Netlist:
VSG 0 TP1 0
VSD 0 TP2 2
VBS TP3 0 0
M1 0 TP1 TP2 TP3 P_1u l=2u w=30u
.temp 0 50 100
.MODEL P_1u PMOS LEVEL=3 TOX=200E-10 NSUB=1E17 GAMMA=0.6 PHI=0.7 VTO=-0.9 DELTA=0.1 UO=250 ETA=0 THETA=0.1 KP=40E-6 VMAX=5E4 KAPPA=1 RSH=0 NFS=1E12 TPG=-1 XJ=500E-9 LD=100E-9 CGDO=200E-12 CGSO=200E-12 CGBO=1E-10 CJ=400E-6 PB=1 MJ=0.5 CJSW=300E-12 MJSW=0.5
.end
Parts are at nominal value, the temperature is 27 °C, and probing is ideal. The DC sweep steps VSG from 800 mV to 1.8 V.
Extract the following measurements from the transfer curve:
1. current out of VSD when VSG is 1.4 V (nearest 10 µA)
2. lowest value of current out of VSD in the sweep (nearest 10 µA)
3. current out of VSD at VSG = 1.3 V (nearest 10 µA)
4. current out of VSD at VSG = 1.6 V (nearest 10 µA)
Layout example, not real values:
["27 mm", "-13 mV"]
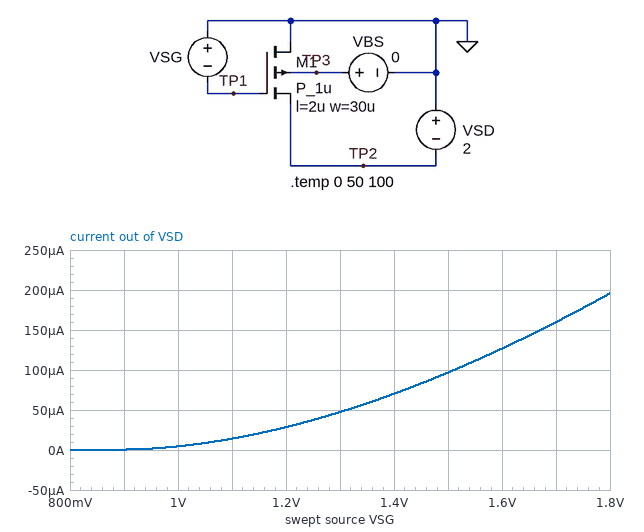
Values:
["70 µA", "0 A", "50 µA", "130 µA"]
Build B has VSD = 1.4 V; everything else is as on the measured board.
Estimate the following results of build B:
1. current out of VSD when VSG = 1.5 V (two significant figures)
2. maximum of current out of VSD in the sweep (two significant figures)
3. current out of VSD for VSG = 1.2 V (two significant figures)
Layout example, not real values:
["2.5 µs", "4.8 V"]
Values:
["96 µA", "190 µA", "28 µA"]
